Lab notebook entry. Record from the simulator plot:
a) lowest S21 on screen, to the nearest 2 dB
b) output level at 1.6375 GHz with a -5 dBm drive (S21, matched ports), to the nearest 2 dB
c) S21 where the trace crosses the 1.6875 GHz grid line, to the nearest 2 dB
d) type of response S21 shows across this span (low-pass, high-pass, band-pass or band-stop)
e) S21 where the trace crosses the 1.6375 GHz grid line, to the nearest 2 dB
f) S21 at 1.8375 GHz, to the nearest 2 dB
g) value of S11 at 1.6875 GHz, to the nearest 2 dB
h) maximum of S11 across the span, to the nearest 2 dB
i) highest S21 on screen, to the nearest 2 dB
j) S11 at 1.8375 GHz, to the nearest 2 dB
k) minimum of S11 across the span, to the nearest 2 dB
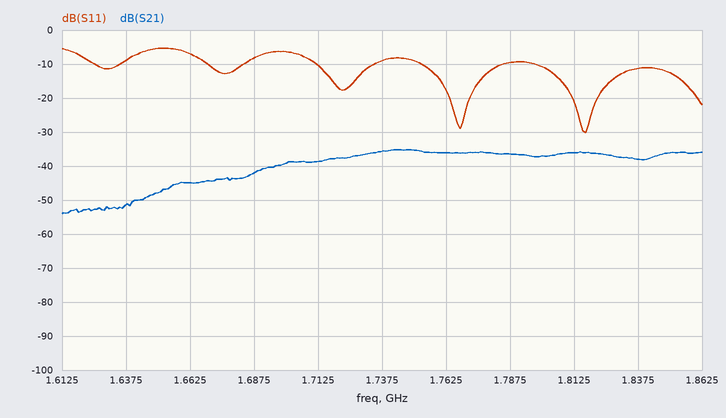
-54 dB
-56 dBm
-42 dB
high-pass
-52 dB
-38 dB
-8 dB
-6 dB
-36 dB
-12 dB
-30 dB
